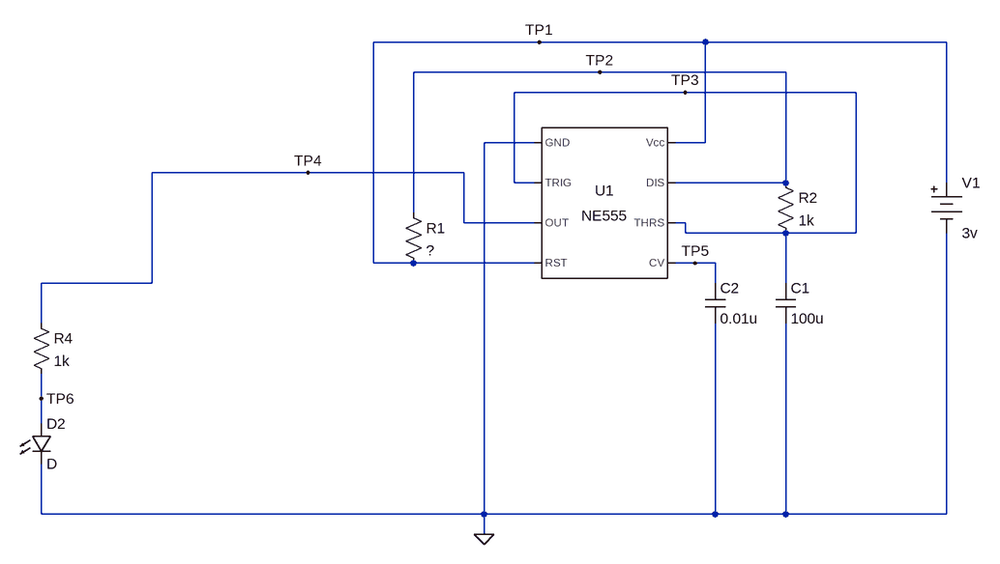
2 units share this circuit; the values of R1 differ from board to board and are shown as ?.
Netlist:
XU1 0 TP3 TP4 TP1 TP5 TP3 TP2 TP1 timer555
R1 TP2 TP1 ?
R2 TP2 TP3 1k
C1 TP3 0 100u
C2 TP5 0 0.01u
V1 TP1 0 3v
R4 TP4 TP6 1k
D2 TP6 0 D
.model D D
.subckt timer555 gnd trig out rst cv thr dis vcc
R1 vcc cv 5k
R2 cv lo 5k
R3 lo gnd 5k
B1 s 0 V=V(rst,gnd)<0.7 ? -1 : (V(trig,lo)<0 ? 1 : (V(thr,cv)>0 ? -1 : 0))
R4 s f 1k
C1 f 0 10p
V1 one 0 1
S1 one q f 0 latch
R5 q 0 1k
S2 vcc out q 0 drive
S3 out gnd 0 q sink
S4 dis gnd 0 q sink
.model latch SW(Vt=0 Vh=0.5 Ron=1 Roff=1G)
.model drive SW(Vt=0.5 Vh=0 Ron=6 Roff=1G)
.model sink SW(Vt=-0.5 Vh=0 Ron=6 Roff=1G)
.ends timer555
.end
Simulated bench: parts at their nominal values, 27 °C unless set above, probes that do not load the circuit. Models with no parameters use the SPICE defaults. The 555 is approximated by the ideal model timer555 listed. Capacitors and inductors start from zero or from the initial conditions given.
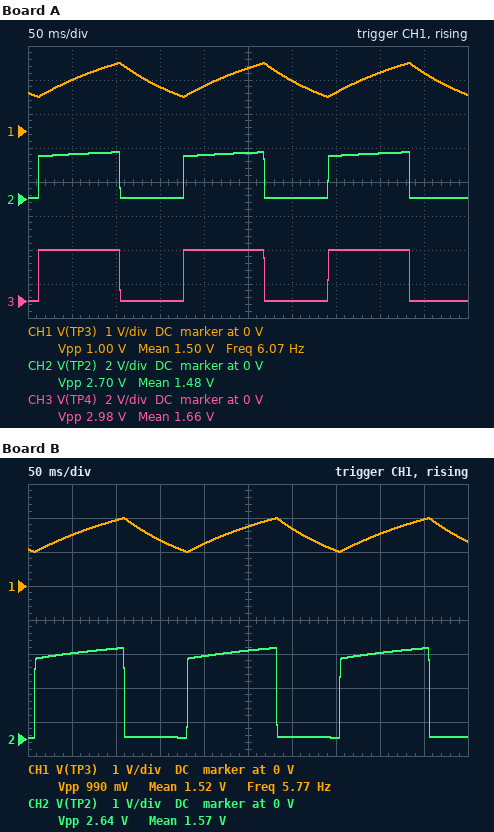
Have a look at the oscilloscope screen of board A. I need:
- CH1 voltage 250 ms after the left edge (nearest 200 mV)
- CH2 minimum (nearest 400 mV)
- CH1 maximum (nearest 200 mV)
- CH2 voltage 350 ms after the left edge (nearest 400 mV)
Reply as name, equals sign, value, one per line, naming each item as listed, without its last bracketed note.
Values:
CH1 voltage 250 ms after the left edge = 1.8 V
CH2 minimum = 0 V
CH1 maximum = 2.0 V
CH2 voltage 350 ms after the left edge = 2.4 V
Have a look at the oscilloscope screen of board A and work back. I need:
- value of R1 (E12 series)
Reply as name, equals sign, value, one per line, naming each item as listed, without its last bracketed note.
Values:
value of R1 = 330 Ω
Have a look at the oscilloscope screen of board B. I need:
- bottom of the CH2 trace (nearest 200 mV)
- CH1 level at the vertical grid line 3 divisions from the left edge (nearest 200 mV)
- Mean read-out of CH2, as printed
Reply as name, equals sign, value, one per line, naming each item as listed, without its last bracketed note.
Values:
bottom of the CH2 trace = 0 V
CH1 level at the vertical grid line 3 divisions from the left edge = 1.4 V
Mean read-out of CH2, as printed = 1.57 V
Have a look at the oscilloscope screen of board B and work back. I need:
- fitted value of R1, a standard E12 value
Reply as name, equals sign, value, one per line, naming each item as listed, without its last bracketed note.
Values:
fitted value of R1, a standard E12 value = 470 Ω
